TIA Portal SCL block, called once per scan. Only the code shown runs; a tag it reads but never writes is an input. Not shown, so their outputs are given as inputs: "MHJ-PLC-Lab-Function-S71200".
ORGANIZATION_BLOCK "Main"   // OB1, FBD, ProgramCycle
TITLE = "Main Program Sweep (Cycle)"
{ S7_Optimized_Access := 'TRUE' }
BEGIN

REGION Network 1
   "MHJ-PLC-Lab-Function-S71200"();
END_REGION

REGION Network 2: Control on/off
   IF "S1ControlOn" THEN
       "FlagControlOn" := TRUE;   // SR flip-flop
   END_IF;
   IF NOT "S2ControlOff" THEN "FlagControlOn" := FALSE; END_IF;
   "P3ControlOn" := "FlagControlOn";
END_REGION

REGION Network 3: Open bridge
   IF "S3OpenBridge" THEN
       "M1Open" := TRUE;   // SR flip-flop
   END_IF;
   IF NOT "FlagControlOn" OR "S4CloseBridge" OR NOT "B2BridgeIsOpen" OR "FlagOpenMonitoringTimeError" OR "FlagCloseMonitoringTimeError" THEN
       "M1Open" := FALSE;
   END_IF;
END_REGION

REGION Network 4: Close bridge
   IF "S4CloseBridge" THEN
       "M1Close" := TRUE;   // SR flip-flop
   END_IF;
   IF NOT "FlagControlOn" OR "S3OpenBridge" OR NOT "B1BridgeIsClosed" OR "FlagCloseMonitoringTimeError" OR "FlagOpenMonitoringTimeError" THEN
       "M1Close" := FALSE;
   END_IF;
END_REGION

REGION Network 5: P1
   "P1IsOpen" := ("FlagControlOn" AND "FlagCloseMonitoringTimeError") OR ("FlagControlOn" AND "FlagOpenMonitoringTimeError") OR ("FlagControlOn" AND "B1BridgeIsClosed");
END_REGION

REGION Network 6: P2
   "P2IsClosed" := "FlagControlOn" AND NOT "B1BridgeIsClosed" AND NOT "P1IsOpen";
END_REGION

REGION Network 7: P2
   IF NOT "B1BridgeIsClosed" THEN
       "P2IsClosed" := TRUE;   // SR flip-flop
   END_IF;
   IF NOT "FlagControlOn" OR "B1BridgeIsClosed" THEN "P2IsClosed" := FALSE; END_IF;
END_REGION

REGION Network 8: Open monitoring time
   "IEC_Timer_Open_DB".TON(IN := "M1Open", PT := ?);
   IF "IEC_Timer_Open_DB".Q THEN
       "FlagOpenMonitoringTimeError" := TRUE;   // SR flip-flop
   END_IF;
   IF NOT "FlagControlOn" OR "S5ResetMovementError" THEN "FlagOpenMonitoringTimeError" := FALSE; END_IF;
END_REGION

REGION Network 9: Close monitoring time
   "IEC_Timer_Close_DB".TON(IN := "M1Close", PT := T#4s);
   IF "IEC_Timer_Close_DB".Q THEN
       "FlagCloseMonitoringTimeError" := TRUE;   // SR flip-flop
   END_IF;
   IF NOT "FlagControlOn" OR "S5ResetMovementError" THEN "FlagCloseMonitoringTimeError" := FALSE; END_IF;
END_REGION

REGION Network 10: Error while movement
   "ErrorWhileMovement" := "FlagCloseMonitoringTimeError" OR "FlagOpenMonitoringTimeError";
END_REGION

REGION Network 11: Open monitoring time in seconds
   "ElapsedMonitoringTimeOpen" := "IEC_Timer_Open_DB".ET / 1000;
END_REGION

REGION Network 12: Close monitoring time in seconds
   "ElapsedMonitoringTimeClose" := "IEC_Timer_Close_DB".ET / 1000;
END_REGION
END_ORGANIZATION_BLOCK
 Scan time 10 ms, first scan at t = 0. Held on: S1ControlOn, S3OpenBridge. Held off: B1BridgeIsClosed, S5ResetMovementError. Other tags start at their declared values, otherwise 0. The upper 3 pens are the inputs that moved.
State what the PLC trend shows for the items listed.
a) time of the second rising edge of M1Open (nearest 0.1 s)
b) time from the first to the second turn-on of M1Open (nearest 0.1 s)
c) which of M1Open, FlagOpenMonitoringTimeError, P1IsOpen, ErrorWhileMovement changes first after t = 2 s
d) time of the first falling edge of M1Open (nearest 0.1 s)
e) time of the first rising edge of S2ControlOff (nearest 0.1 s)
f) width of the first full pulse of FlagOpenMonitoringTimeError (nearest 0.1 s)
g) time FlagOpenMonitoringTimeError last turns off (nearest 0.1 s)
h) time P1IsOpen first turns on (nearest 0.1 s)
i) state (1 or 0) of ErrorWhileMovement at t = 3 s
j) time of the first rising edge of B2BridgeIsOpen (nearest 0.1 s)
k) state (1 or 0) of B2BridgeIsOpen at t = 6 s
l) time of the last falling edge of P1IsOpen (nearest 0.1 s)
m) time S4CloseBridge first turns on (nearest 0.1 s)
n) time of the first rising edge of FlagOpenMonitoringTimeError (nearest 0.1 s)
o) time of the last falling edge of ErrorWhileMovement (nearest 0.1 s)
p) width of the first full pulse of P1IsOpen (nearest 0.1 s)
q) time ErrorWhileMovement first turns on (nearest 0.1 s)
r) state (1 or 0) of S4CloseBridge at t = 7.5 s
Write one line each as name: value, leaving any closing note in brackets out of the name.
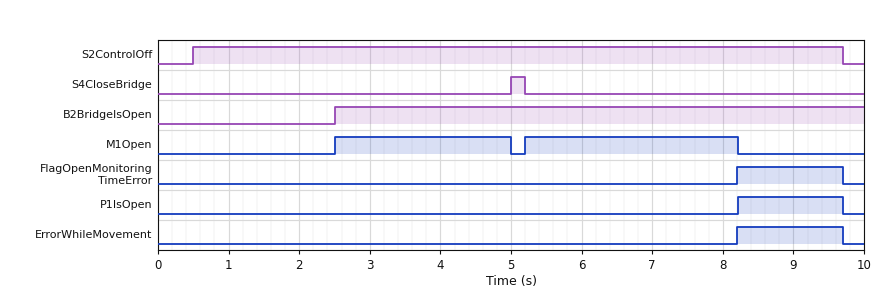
time of the second rising edge of M1Open: 5.2 s
time from the first to the second turn-on of M1Open: 2.7 s
which of M1Open, FlagOpenMonitoringTimeError, P1IsOpen, ErrorWhileMovement changes first after t = 2 s: M1Open
time of the first falling edge of M1Open: 5.0 s
time of the first rising edge of S2ControlOff: 0.5 s
width of the first full pulse of FlagOpenMonitoringTimeError: 1.5 s
time FlagOpenMonitoringTimeError last turns off: 9.7 s
time P1IsOpen first turns on: 8.2 s
state (1 or 0) of ErrorWhileMovement at t = 3 s: 0
time of the first rising edge of B2BridgeIsOpen: 2.5 s
state (1 or 0) of B2BridgeIsOpen at t = 6 s: 1
time of the last falling edge of P1IsOpen: 9.7 s
time S4CloseBridge first turns on: 5.0 s
time of the first rising edge of FlagOpenMonitoringTimeError: 8.2 s
time of the last falling edge of ErrorWhileMovement: 9.7 s
width of the first full pulse of P1IsOpen: 1.5 s
time ErrorWhileMovement first turns on: 8.2 s
state (1 or 0) of S4CloseBridge at t = 7.5 s: 0
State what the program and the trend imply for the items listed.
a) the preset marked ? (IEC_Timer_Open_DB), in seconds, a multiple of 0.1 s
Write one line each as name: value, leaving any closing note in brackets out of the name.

the preset marked ? (IEC_Timer_Open_DB), in seconds, a multiple of 0.1 s: 3.0 s
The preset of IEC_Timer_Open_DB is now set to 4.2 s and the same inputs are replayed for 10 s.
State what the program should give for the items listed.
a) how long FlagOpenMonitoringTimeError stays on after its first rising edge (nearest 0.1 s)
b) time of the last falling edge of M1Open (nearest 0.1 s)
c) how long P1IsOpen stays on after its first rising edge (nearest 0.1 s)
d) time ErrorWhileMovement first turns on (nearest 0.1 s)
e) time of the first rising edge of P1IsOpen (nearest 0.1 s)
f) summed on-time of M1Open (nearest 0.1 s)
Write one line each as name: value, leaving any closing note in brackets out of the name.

how long FlagOpenMonitoringTimeError stays on after its first rising edge: 0.3 s
time of the last falling edge of M1Open: 9.4 s
how long P1IsOpen stays on after its first rising edge: 0.3 s
time ErrorWhileMovement first turns on: 9.4 s
time of the first rising edge of P1IsOpen: 9.4 s
summed on-time of M1Open: 6.7 s
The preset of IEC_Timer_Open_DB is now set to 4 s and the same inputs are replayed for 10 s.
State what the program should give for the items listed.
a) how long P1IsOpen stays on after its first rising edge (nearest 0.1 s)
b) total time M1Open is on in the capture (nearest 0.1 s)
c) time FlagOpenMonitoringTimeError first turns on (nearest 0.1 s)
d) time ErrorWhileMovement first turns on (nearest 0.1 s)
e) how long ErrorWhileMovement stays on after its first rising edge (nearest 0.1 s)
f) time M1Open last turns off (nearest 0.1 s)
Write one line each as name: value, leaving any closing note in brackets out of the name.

how long P1IsOpen stays on after its first rising edge: 0.5 s
total time M1Open is on in the capture: 6.5 s
time FlagOpenMonitoringTimeError first turns on: 9.2 s
time ErrorWhileMovement first turns on: 9.2 s
how long ErrorWhileMovement stays on after its first rising edge: 0.5 s
time M1Open last turns off: 9.2 s
